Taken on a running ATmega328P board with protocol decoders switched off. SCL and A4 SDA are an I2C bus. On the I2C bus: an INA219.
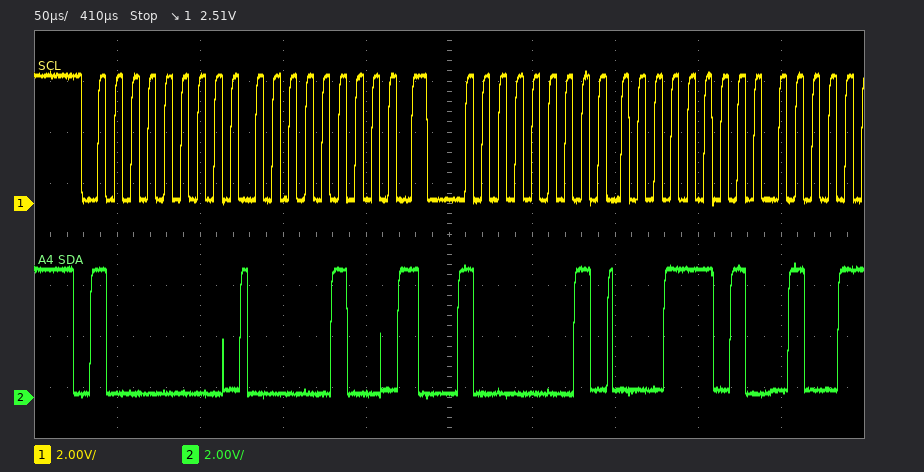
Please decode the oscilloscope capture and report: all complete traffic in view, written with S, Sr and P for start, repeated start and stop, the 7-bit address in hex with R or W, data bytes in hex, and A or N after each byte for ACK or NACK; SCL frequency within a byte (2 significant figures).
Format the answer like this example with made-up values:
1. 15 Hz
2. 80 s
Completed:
1. S 40W A 04 A Sr 40R A 1D A
2. 100 kHz
